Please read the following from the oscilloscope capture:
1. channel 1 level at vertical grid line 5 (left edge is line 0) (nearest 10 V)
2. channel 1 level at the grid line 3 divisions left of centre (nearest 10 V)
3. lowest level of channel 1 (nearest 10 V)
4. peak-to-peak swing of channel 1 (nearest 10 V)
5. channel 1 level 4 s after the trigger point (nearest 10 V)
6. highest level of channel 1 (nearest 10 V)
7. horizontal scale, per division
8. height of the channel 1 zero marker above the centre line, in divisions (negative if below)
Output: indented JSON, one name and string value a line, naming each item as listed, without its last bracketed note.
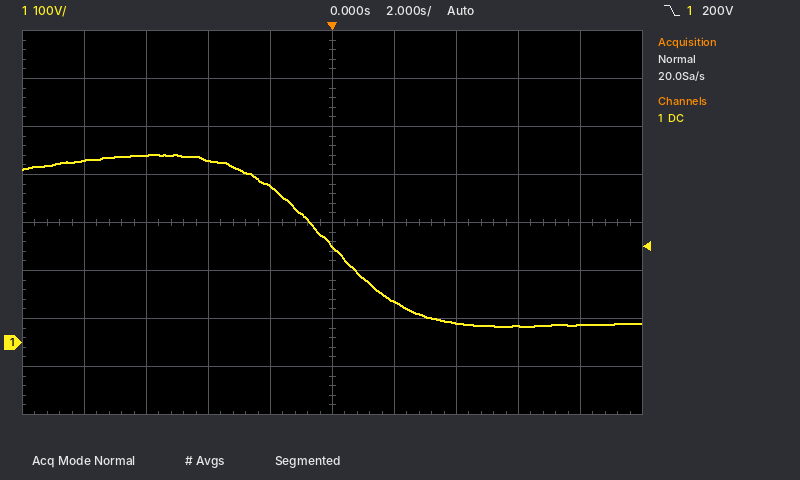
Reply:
{
  "channel 1 level at vertical grid line 5 (left edge is line 0)": "200 V",
  "channel 1 level at the grid line 3 divisions left of centre": "390 V",
  "lowest level of channel 1": "30 V",
  "peak-to-peak swing of channel 1": "360 V",
  "channel 1 level 4 s after the trigger point": "40 V",
  "highest level of channel 1": "390 V",
  "horizontal scale, per division": "2 s",
  "height of the channel 1 zero marker above the centre line, in divisions": "-2.5 div"
}
